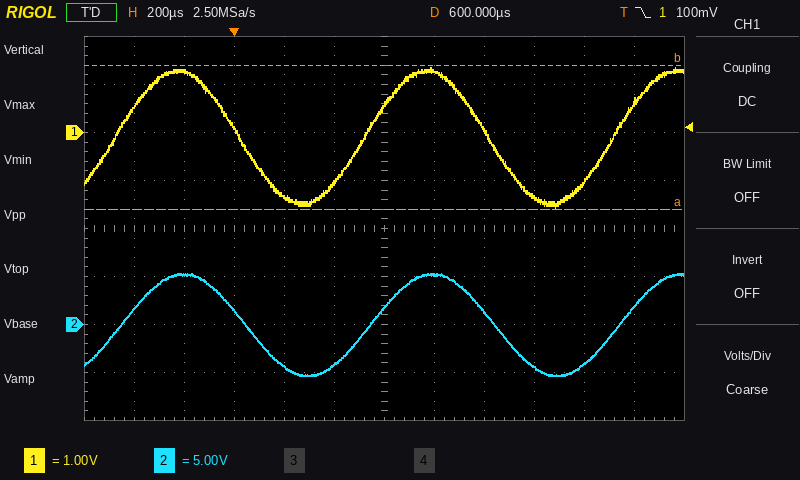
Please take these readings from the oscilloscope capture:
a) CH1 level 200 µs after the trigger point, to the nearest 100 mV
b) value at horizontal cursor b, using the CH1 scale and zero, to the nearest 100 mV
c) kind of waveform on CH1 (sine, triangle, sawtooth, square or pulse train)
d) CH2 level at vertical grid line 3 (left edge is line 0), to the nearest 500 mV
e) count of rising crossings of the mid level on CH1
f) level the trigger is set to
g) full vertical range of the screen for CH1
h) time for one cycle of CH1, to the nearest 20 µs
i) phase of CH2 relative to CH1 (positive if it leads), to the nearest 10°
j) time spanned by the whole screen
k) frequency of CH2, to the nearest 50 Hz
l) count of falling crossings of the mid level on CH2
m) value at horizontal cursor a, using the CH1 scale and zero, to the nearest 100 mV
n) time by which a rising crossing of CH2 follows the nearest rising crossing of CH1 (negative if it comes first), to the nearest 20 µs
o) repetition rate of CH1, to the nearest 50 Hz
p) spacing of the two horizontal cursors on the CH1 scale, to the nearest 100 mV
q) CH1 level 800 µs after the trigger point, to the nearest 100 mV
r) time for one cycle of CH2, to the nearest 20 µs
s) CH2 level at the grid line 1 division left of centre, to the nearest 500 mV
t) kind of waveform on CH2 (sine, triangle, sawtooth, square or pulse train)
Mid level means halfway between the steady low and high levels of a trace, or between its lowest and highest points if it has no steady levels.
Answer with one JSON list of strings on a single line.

["-1.3 V", "1.4 V", "sine", "1.5 V", "3", "100 mV", "8 V", "1.00 ms", "-10°", "2.4 ms", "1.00 kHz", "2", "-1.6 V", "+20 µs", "1.00 kHz", "3.0 V", "1.3 V", "1.00 ms", "-4.0 V", "sine"]
